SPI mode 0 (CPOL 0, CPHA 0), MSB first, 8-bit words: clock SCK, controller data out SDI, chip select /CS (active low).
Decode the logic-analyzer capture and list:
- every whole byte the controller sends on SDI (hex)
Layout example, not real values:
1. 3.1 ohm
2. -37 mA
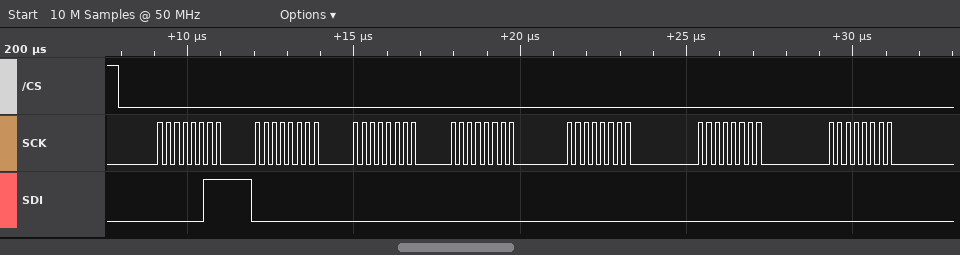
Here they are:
1. 03 00 00 00 00 00 00
